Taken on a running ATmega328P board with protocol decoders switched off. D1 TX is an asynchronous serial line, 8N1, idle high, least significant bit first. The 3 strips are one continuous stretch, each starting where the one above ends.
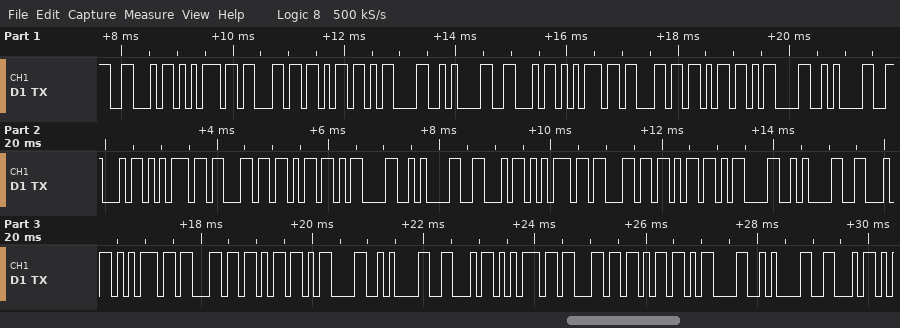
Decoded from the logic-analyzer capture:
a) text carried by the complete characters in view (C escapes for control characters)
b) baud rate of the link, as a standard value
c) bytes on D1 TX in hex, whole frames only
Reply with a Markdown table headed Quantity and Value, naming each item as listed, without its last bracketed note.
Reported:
| Quantity | Value |
|---|---|
| text carried by the complete characters in view | "Fuck\r\nFuck\r\nFuck\r\nFuck\r\nFuck\r\nFuck\r\nF" |
| baud rate of the link, as a standard value | 9600 baud |
| bytes on D1 TX in hex, whole frames only | 0x46 0x75 0x63 0x6B 0x0D 0x0A 0x46 0x75 0x63 0x6B 0x0D 0x0A 0x46 0x75 0x63 0x6B 0x0D 0x0A 0x46 0x75 0x63 0x6B 0x0D 0x0A 0x46 0x75 0x63 0x6B 0x0D 0x0A 0x46 0x75 0x63 0x6B 0x0D 0x0A 0x46 |
